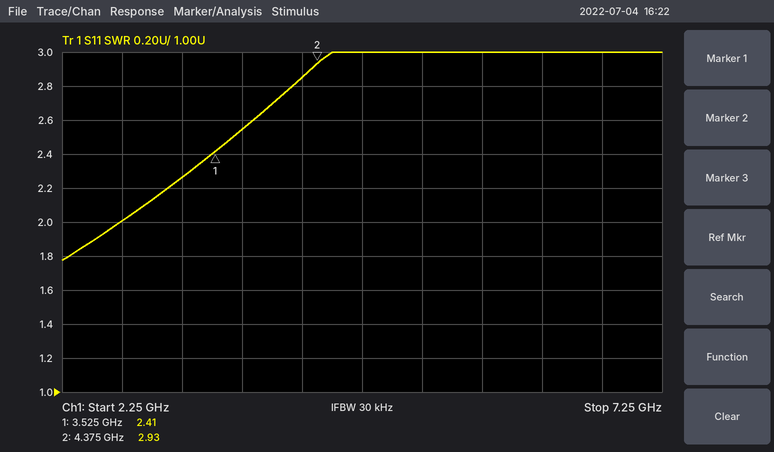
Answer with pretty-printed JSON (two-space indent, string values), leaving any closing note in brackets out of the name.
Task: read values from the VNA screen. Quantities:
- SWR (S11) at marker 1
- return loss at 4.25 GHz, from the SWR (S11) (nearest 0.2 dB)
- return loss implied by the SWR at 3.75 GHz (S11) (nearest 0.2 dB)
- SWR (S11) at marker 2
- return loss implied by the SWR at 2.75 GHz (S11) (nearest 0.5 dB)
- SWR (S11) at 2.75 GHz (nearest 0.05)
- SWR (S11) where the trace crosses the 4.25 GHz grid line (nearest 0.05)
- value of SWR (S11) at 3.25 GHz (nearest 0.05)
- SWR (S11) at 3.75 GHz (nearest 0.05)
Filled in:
{
  "SWR (S11) at marker 1": "2.41",
  "return loss at 4.25 GHz, from the SWR (S11)": "6.4 dB",
  "return loss implied by the SWR at 3.75 GHz (S11)": "7.2 dB",
  "SWR (S11) at marker 2": "2.93",
  "return loss implied by the SWR at 2.75 GHz (S11)": "9.5 dB",
  "SWR (S11) at 2.75 GHz": "2.00",
  "SWR (S11) where the trace crosses the 4.25 GHz grid line": "2.85",
  "value of SWR (S11) at 3.25 GHz": "2.25",
  "SWR (S11) at 3.75 GHz": "2.55"
}
